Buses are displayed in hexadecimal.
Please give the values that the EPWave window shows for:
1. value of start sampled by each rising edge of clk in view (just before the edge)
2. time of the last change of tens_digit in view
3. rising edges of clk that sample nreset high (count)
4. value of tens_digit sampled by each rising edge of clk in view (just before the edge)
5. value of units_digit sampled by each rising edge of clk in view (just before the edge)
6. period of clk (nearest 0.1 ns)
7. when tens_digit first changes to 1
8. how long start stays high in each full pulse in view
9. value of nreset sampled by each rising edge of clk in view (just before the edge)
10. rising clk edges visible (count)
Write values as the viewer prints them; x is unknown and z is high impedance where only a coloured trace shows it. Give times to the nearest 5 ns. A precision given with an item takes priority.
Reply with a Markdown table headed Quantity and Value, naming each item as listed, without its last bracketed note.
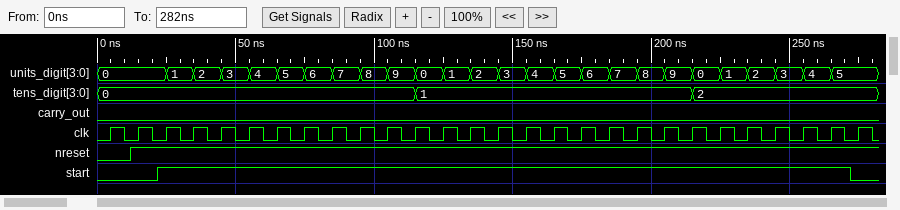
| Quantity | Value |
|---|---|
| value of start sampled by each rising edge of clk in view | 0 0 1 1 1 1 1 1 1 1 1 1 1 1 1 1 1 1 1 1 1 1 1 1 1 1 1 0 |
| time of the last change of tens_digit in view | 215 ns |
| rising edges of clk that sample nreset high | 27 |
| value of tens_digit sampled by each rising edge of clk in view | 0, 0, 0, 0, 0, 0, 0, 0, 0, 0, 0, 0, 1, 1, 1, 1, 1, 1, 1, 1, 1, 1, 2, 2, 2, 2, 2, 2 |
| value of units_digit sampled by each rising edge of clk in view | 0, 0, 0, 1, 2, 3, 4, 5, 6, 7, 8, 9, 0, 1, 2, 3, 4, 5, 6, 7, 8, 9, 0, 1, 2, 3, 4, 5 |
| period of clk | 10 ns |
| when tens_digit first changes to 1 | 115 ns |
| how long start stays high in each full pulse in view | 250 ns |
| value of nreset sampled by each rising edge of clk in view | 0 1 1 1 1 1 1 1 1 1 1 1 1 1 1 1 1 1 1 1 1 1 1 1 1 1 1 1 |
| rising clk edges visible | 28 |
